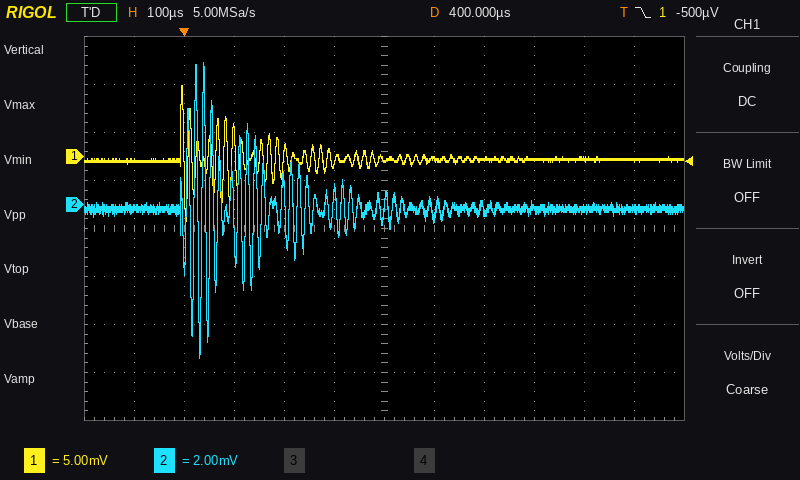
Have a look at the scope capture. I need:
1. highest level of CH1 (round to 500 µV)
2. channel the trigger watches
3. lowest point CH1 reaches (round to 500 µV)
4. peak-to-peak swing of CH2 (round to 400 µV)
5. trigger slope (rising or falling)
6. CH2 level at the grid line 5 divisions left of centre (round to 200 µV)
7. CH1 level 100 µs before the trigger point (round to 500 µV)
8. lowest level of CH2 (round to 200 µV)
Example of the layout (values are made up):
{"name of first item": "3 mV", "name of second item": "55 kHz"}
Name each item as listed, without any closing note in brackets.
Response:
{"highest level of CH1": "7.5 mV", "channel the trigger watches": "CH1", "lowest point CH1 reaches": "-7.0 mV", "peak-to-peak swing of CH2": "12.4 mV", "trigger slope": "falling", "CH2 level at the grid line 5 divisions left of centre": "-200 µV", "CH1 level 100 µs before the trigger point": "-500 µV", "lowest level of CH2": "-6.4 mV"}
